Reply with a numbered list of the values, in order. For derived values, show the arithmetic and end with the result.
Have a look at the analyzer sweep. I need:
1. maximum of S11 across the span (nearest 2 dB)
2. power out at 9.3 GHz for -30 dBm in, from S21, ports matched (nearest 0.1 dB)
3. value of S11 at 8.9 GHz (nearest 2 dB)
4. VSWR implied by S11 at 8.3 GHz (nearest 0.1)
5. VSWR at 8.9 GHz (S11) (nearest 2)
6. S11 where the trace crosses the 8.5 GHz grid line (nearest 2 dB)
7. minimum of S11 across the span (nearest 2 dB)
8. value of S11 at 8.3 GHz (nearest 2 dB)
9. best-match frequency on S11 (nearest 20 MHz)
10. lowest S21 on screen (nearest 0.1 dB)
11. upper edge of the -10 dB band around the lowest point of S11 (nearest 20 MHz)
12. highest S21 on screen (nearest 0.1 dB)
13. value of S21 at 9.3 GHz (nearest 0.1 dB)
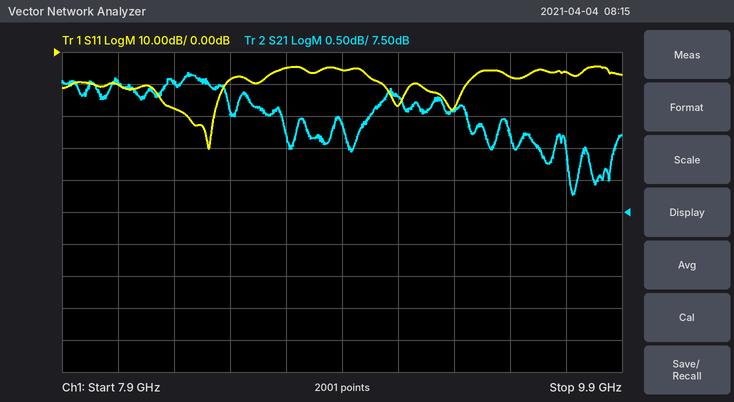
1. -4 dB
2. -30 dBm + (9.1 dB) = -20.9 dBm
3. -6 dB
4. |Γ| = 10^(-18/20) = 0.1259; VSWR = (1 + 0.1259)/(1 − 0.1259) ≈ 1.3
5. |Γ| = 10^(-6/20) = 0.5012; VSWR = (1 + 0.5012)/(1 − 0.5012) ≈ 3.01, so 4 to the nearest 2
6. -8 dB
7. -30 dB
8. -18 dB
9. 8.42 GHz
10. 7.8 dB
11. 8.48 GHz
12. 9.7 dB
13. 9.1 dB
